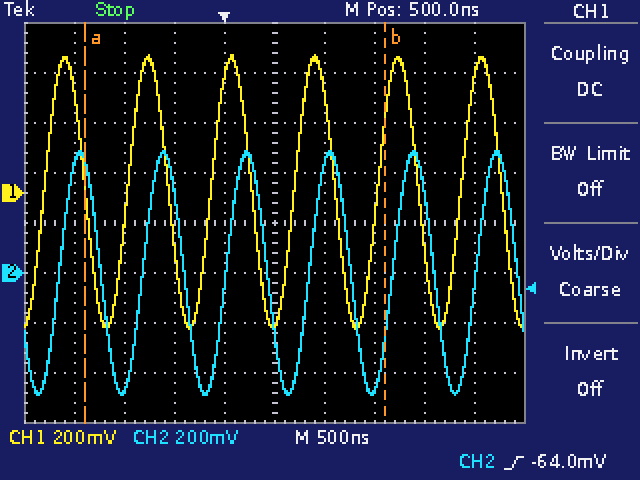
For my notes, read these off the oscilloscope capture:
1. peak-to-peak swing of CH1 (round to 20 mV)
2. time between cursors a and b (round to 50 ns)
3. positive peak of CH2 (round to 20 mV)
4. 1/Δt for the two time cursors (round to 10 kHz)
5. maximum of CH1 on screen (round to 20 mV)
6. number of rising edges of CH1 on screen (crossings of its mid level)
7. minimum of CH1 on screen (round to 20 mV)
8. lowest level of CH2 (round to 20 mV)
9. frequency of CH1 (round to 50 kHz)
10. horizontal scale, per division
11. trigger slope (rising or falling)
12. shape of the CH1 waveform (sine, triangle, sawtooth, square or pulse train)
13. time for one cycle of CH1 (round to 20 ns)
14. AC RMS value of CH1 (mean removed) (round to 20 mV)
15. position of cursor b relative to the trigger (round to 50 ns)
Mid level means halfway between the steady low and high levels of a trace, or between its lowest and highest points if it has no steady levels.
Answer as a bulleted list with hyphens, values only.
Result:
- 1.10 V
- 3.00 µs
- 480 mV
- 330 kHz
- 560 mV
- 6
- -540 mV
- -480 mV
- 1.20 MHz
- 500 ns
- rising
- sine
- 840 ns
- 380 mV
- +1.60 µs
